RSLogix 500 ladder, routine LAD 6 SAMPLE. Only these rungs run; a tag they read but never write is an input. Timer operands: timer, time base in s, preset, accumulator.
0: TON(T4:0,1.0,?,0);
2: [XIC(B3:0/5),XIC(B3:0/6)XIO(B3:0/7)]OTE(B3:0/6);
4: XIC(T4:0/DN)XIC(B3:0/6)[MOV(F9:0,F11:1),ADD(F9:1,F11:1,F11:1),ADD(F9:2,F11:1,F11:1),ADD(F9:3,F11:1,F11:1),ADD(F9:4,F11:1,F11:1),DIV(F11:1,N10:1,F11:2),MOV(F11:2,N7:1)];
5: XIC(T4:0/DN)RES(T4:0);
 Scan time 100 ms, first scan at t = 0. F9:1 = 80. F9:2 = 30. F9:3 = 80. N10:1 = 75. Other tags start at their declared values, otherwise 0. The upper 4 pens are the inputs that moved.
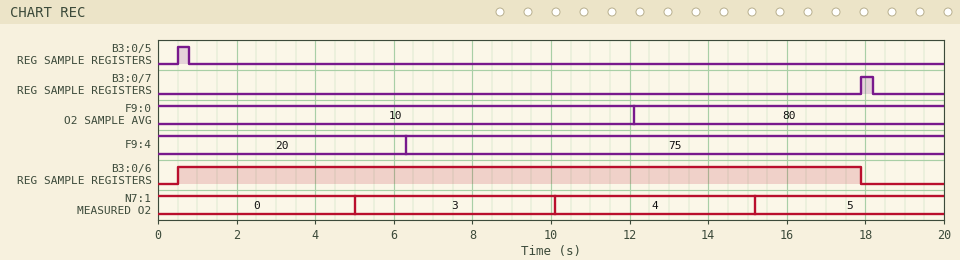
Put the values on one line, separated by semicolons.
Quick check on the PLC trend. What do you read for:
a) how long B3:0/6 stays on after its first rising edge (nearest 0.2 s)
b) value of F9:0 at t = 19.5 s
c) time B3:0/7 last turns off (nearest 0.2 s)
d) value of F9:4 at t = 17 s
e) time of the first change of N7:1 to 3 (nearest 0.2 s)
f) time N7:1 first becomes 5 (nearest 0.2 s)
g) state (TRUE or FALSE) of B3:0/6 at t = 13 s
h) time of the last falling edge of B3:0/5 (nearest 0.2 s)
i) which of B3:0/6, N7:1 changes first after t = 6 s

17.4 s; 80; 18.2 s; 75; 5.0 s; 15.2 s; TRUE; 0.8 s; N7:1
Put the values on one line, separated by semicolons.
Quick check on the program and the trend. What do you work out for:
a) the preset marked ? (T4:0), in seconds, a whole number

5 s
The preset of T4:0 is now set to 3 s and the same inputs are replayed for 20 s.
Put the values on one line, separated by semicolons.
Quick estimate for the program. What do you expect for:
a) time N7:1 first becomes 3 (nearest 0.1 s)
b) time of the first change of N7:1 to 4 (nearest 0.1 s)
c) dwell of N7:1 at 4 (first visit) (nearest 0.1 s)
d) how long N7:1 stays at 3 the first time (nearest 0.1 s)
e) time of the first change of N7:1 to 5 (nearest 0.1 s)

3.0 s; 9.2 s; 3.1 s; 6.2 s; 12.3 s
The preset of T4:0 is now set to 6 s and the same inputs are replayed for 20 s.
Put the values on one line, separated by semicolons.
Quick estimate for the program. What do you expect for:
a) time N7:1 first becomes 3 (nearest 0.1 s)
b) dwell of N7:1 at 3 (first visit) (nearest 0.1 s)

6.0 s; 6.1 s
